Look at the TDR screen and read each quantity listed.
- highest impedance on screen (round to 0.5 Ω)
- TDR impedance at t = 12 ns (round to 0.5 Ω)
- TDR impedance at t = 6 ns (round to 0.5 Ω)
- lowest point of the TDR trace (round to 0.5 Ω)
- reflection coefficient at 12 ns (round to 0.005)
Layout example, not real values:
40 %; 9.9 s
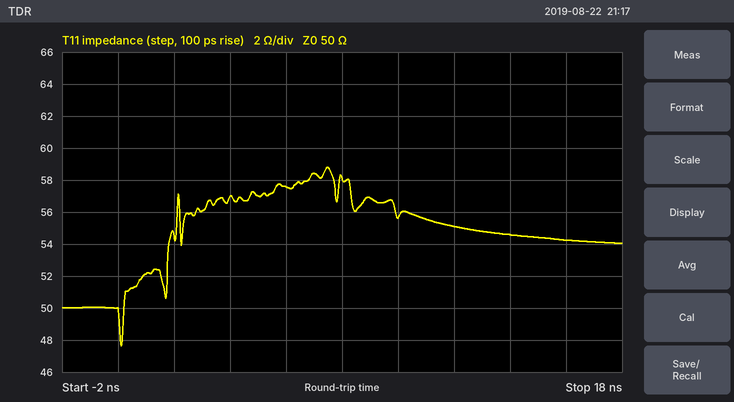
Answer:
59.0 Ω; 55.0 Ω; 57.5 Ω; 47.5 Ω; +0.050
